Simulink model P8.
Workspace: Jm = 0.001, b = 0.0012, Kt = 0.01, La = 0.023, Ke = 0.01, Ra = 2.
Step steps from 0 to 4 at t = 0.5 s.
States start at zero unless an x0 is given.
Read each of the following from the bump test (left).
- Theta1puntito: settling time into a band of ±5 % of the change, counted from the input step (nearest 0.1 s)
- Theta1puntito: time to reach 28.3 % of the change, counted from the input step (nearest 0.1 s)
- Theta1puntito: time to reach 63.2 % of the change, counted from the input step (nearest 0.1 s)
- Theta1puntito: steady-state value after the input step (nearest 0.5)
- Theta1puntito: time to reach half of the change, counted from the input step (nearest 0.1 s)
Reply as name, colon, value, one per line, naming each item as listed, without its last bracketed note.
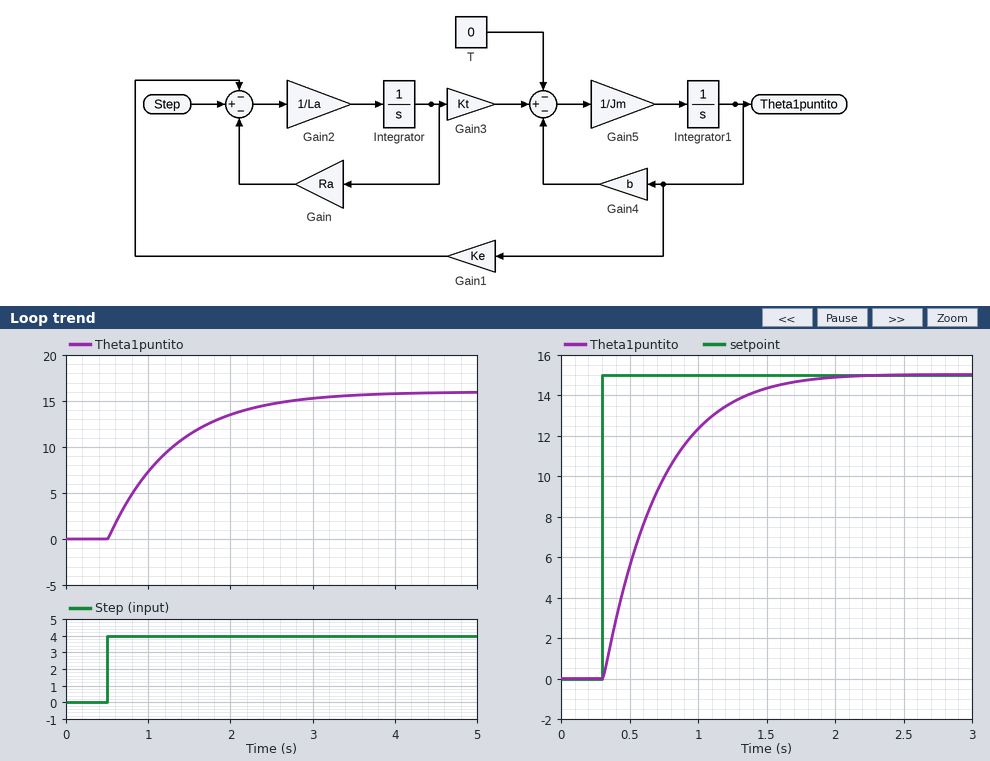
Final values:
Theta1puntito: settling time into a band of ±5 % of the change, counted from the input step: 2.4 s
Theta1puntito: time to reach 28.3 % of the change, counted from the input step: 0.3 s
Theta1puntito: time to reach 63.2 % of the change, counted from the input step: 0.8 s
Theta1puntito: steady-state value after the input step: 16.0
Theta1puntito: time to reach half of the change, counted from the input step: 0.6 s
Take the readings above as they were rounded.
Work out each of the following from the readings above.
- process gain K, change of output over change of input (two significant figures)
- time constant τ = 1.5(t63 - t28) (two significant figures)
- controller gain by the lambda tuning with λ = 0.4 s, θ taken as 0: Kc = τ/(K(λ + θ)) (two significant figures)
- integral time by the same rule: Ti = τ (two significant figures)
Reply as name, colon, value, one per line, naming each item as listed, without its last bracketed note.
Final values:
process gain K, change of output over change of input: 4.0
time constant τ = 1.5(t63 - t28): 0.75 s
controller gain by the lambda tuning with λ = 0.4 s, θ taken as 0: Kc = τ/(K(λ + θ)): 0.47
integral time by the same rule: Ti = τ: 0.75 s
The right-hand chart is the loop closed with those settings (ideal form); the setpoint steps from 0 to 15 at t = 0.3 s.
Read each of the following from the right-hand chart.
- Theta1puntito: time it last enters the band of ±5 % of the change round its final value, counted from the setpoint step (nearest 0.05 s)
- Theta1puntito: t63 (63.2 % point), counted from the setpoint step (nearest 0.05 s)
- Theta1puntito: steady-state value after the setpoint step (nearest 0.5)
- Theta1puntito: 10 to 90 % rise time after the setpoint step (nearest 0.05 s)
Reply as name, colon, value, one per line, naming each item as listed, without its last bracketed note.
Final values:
Theta1puntito: time it last enters the band of ±5 % of the change round its final value, counted from the setpoint step: 1.15 s
Theta1puntito: t63 (63.2 % point), counted from the setpoint step: 0.40 s
Theta1puntito: steady-state value after the setpoint step: 15.0
Theta1puntito: 10 to 90 % rise time after the setpoint step: 0.85 s
